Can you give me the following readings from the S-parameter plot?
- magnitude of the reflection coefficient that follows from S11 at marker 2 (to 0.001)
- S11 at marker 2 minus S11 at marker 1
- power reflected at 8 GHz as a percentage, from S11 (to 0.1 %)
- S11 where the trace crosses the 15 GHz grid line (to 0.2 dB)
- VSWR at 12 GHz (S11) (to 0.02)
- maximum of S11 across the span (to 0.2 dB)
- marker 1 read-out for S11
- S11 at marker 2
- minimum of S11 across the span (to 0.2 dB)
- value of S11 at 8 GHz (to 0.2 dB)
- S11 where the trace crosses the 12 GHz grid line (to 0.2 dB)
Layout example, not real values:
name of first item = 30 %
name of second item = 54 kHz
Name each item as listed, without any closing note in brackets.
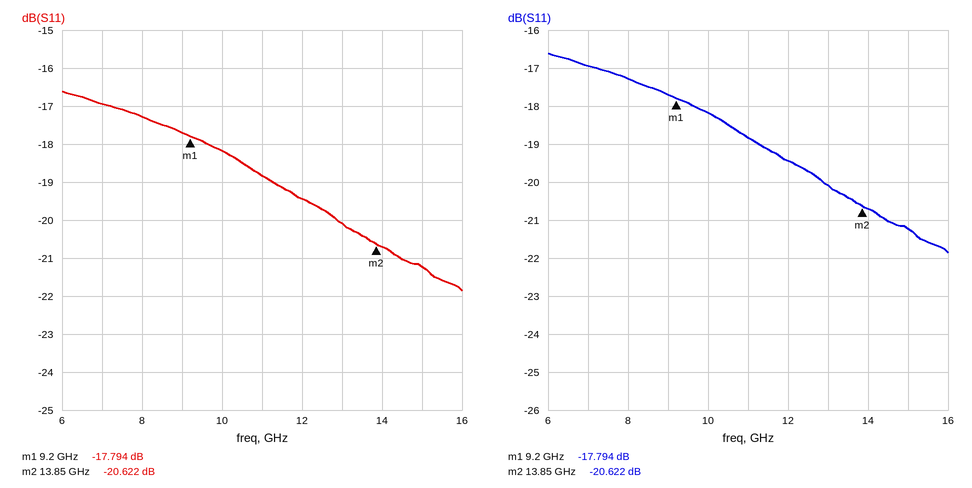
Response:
magnitude of the reflection coefficient that follows from S11 at marker 2 = 0.093
S11 at marker 2 minus S11 at marker 1 = -2.828 dB
power reflected at 8 GHz as a percentage, from S11 = 1.9 %
S11 where the trace crosses the 15 GHz grid line = -21.2 dB
VSWR at 12 GHz (S11) = 1.24
maximum of S11 across the span = -16.6 dB
marker 1 read-out for S11 = -17.794 dB
S11 at marker 2 = -20.622 dB
minimum of S11 across the span = -21.8 dB
value of S11 at 8 GHz = -17.2 dB
S11 where the trace crosses the 12 GHz grid line = -19.4 dB
